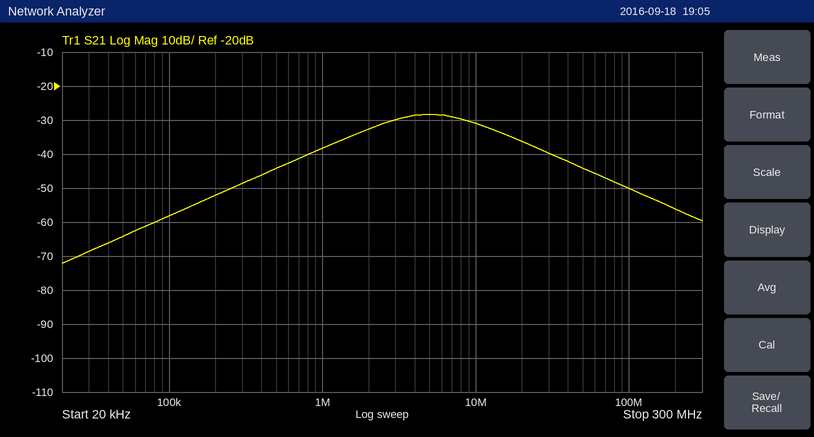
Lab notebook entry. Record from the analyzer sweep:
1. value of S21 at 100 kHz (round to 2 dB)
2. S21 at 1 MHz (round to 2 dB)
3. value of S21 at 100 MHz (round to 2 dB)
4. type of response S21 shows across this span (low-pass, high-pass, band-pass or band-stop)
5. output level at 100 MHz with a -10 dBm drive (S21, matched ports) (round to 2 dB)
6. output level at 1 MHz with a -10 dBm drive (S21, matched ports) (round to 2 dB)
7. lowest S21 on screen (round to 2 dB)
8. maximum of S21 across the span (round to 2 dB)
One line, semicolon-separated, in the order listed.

-58 dB; -38 dB; -50 dB; band-pass; -60 dBm; -48 dBm; -72 dB; -28 dB
